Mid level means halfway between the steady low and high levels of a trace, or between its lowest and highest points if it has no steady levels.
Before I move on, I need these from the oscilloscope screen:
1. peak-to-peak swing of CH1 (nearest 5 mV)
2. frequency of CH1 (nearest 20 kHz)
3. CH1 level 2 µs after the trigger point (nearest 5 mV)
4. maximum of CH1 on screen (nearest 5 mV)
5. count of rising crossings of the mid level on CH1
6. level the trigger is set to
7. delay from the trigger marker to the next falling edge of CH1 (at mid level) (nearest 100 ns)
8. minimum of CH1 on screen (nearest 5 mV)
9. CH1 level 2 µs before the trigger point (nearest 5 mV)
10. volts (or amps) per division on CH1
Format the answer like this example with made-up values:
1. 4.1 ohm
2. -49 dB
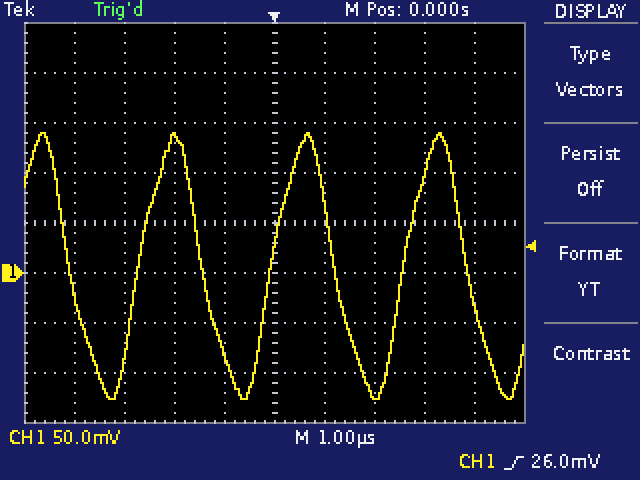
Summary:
1. 265 mV
2. 380 kHz
3. -120 mV
4. 140 mV
5. 3
6. 26.0 mV
7. 1.2 µs
8. -125 mV
9. 135 mV
10. 50 mV
